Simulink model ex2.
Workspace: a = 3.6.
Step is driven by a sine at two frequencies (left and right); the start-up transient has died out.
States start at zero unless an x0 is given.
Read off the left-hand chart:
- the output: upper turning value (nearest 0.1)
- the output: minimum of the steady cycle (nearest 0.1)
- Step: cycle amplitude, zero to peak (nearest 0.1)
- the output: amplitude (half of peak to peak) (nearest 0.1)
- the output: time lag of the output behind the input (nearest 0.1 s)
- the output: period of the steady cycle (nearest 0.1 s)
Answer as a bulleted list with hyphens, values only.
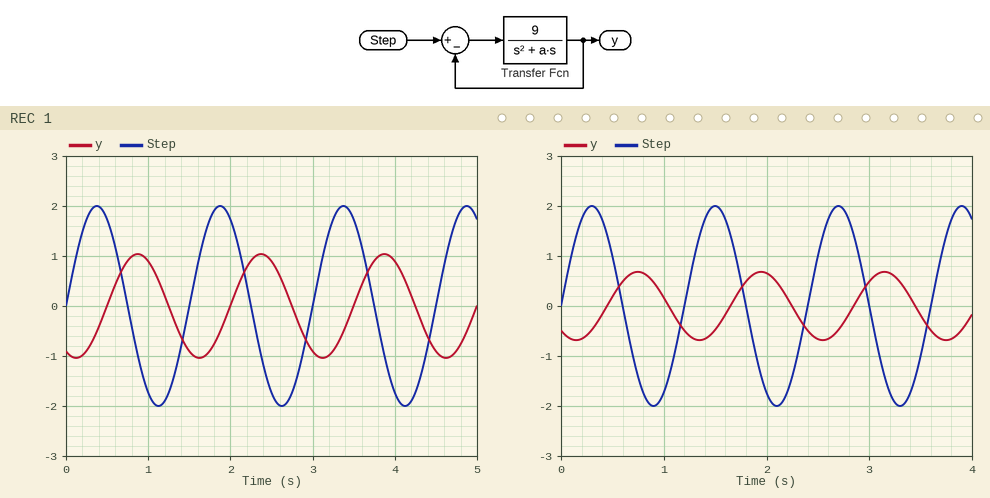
- 1.0
- -1.0
- 2.0
- 1.0
- 0.5 s
- 1.5 s
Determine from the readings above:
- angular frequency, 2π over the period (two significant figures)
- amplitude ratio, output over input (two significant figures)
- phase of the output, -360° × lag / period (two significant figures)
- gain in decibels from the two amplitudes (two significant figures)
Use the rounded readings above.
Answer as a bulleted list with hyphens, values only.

- 4.2 rad/s
- 0.50
- -120°
- -6.0 dB
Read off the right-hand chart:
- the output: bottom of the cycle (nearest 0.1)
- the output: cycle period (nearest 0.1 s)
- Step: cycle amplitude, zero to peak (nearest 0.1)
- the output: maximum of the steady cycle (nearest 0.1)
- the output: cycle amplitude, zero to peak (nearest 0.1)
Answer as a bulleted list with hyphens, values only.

- -0.7
- 1.2 s
- 2.0
- 0.7
- 0.7
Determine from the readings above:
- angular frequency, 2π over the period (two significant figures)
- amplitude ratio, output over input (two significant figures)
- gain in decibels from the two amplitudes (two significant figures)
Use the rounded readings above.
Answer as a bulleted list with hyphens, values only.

- 5.2 rad/s
- 0.35
- -9.1 dB
